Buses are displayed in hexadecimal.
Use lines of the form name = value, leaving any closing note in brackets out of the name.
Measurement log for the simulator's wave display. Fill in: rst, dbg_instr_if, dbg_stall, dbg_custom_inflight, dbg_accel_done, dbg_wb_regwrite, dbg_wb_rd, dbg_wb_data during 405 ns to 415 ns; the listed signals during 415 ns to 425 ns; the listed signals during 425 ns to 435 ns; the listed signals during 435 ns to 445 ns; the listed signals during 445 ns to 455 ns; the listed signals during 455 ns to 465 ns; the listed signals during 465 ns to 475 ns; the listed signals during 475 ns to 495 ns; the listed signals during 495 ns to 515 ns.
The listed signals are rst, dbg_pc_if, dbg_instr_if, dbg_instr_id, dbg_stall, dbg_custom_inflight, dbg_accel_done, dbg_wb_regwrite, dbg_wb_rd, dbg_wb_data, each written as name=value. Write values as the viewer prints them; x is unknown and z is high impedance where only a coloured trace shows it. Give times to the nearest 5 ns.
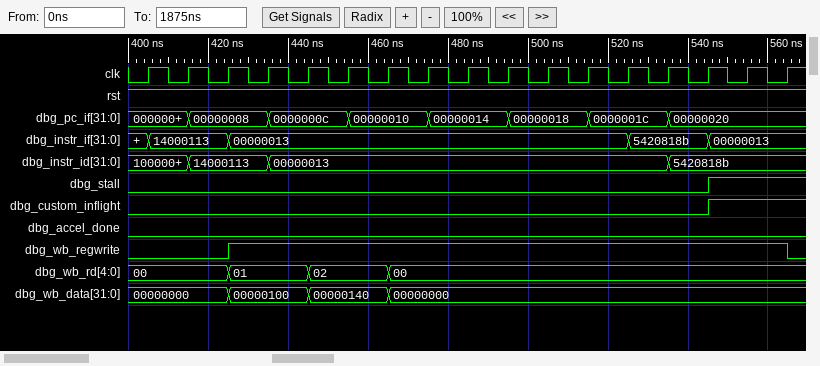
rst, dbg_instr_if, dbg_stall, dbg_custom_inflight, dbg_accel_done, dbg_wb_regwrite, dbg_wb_rd, dbg_wb_data during 405 ns to 415 ns = rst=1, dbg_instr_if=14000113, dbg_stall=0, dbg_custom_inflight=0, dbg_accel_done=0, dbg_wb_regwrite=0, dbg_wb_rd=00, dbg_wb_data=00000000
the listed signals during 415 ns to 425 ns = rst=1, dbg_pc_if=00000008, dbg_instr_if=14000113, dbg_instr_id=14000113, dbg_stall=0, dbg_custom_inflight=0, dbg_accel_done=0, dbg_wb_regwrite=0, dbg_wb_rd=00, dbg_wb_data=00000000
the listed signals during 425 ns to 435 ns = rst=1, dbg_pc_if=00000008, dbg_instr_if=00000013, dbg_instr_id=14000113, dbg_stall=0, dbg_custom_inflight=0, dbg_accel_done=0, dbg_wb_regwrite=1, dbg_wb_rd=01, dbg_wb_data=00000100
the listed signals during 435 ns to 445 ns = rst=1, dbg_pc_if=0000000c, dbg_instr_if=00000013, dbg_instr_id=00000013, dbg_stall=0, dbg_custom_inflight=0, dbg_accel_done=0, dbg_wb_regwrite=1, dbg_wb_rd=01, dbg_wb_data=00000100
the listed signals during 445 ns to 455 ns = rst=1, dbg_pc_if=0000000c, dbg_instr_if=00000013, dbg_instr_id=00000013, dbg_stall=0, dbg_custom_inflight=0, dbg_accel_done=0, dbg_wb_regwrite=1, dbg_wb_rd=02, dbg_wb_data=00000140
the listed signals during 455 ns to 465 ns = rst=1, dbg_pc_if=00000010, dbg_instr_if=00000013, dbg_instr_id=00000013, dbg_stall=0, dbg_custom_inflight=0, dbg_accel_done=0, dbg_wb_regwrite=1, dbg_wb_rd=02, dbg_wb_data=00000140
the listed signals during 465 ns to 475 ns = rst=1, dbg_pc_if=00000010, dbg_instr_if=00000013, dbg_instr_id=00000013, dbg_stall=0, dbg_custom_inflight=0, dbg_accel_done=0, dbg_wb_regwrite=1, dbg_wb_rd=00, dbg_wb_data=00000000
the listed signals during 475 ns to 495 ns = rst=1, dbg_pc_if=00000014, dbg_instr_if=00000013, dbg_instr_id=00000013, dbg_stall=0, dbg_custom_inflight=0, dbg_accel_done=0, dbg_wb_regwrite=1, dbg_wb_rd=00, dbg_wb_data=00000000
the listed signals during 495 ns to 515 ns = rst=1, dbg_pc_if=00000018, dbg_instr_if=00000013, dbg_instr_id=00000013, dbg_stall=0, dbg_custom_inflight=0, dbg_accel_done=0, dbg_wb_regwrite=1, dbg_wb_rd=00, dbg_wb_data=00000000
